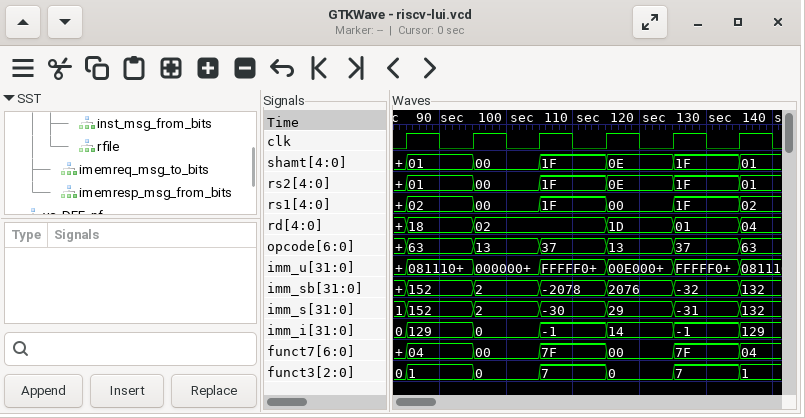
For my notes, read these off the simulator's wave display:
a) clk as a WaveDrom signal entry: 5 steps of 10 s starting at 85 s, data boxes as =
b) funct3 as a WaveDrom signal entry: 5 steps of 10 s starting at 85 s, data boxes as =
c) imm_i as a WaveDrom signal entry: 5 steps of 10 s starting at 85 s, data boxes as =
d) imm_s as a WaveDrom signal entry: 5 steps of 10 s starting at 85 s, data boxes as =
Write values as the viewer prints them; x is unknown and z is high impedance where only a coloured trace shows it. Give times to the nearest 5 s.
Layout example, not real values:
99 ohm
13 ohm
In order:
{name: 'clk', wave: 'p....'}
{name: 'funct3', wave: '=====', data: '1 0 7 0 7'}
{name: 'imm_i', wave: '=====', data: '129 0 -1 14 -1'}
{name: 'imm_s', wave: '=====', data: '152 2 -30 29 -31'}
